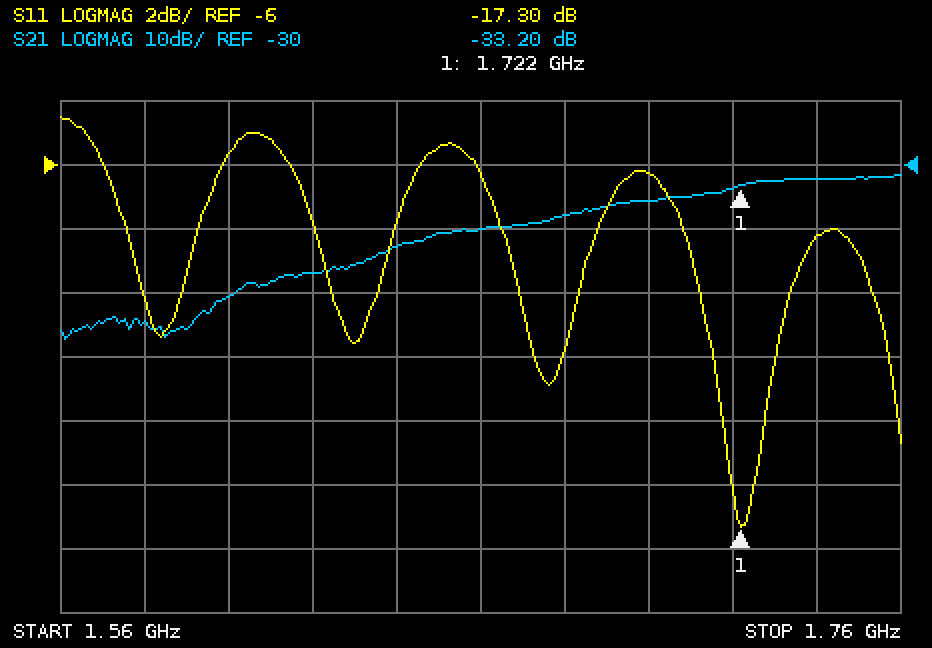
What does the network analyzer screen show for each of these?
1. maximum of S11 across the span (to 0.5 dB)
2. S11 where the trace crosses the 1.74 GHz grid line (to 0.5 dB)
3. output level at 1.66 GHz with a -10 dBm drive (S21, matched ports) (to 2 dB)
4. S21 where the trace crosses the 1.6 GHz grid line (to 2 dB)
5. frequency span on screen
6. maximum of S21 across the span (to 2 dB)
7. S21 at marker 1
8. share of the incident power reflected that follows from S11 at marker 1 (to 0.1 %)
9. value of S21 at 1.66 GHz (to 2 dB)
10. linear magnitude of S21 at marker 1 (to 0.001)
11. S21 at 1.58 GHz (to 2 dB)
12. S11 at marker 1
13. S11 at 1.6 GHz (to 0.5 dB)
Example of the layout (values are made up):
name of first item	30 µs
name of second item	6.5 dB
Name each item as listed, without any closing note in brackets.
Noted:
maximum of S11 across the span	-4.5 dB
S11 where the trace crosses the 1.74 GHz grid line	-8.0 dB
output level at 1.66 GHz with a -10 dBm drive (S21, matched ports)	-50 dBm
S21 where the trace crosses the 1.6 GHz grid line	-50 dB
frequency span on screen	200 MHz
maximum of S21 across the span	-32 dB
S21 at marker 1	-33.20 dB
share of the incident power reflected that follows from S11 at marker 1	1.9 %
value of S21 at 1.66 GHz	-40 dB
linear magnitude of S21 at marker 1	0.022
S21 at 1.58 GHz	-54 dB
S11 at marker 1	-17.30 dB
S11 at 1.6 GHz	-5.5 dB
